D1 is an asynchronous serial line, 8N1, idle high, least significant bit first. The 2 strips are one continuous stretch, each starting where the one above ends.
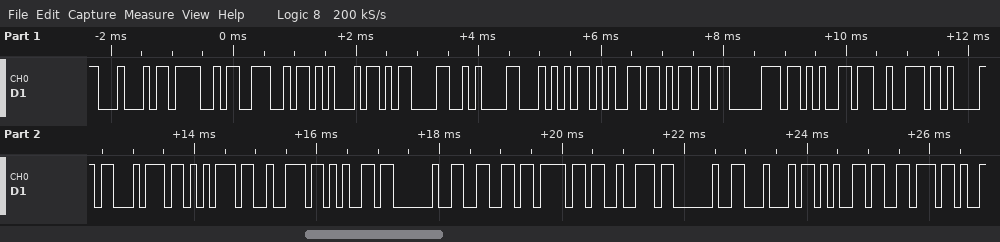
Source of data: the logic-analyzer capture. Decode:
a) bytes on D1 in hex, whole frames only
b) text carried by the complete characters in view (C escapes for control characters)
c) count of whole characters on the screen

44 4F 4E 45 0D 0A 54 65 6D 70 65 72 61 74 75 72 65 20 66 6F 72 20 44 65 76
"DONE\r\nTemperature for Dev"
25
